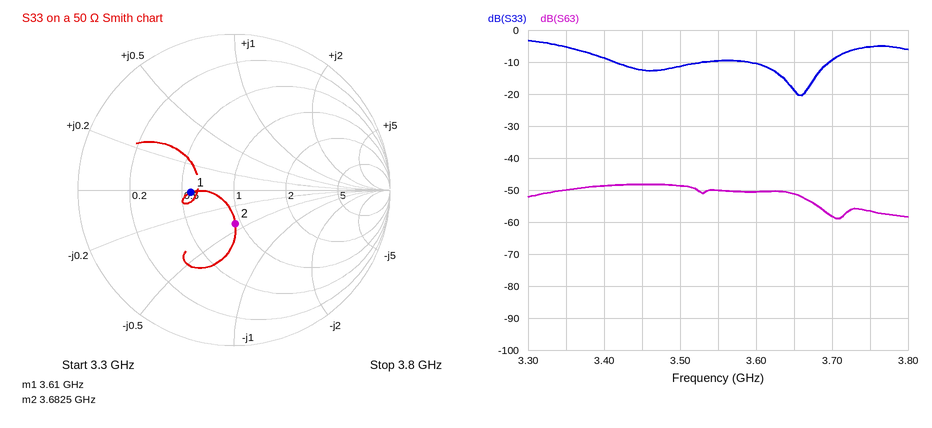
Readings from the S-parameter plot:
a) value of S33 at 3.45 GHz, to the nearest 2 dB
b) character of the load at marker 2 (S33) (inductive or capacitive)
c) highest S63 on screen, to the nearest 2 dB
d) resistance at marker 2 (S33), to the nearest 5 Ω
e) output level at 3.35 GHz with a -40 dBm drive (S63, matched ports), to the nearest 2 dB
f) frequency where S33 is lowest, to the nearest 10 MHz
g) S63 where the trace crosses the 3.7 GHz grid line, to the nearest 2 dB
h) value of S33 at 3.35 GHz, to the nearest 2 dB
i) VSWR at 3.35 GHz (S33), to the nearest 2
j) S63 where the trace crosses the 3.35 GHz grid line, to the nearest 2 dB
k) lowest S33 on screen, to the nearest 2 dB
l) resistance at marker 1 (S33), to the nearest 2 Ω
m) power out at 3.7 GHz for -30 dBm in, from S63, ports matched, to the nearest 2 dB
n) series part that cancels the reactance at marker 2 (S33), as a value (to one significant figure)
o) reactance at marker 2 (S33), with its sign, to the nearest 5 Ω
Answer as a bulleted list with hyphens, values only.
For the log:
- -12 dB
- capacitive
- -48 dB
- 45 Ω
- -90 dBm
- 3.66 GHz
- -58 dB
- -6 dB
- 4
- -50 dB
- -20 dB
- 28 Ω
- -88 dBm
- 900 pH
- -20 Ω
